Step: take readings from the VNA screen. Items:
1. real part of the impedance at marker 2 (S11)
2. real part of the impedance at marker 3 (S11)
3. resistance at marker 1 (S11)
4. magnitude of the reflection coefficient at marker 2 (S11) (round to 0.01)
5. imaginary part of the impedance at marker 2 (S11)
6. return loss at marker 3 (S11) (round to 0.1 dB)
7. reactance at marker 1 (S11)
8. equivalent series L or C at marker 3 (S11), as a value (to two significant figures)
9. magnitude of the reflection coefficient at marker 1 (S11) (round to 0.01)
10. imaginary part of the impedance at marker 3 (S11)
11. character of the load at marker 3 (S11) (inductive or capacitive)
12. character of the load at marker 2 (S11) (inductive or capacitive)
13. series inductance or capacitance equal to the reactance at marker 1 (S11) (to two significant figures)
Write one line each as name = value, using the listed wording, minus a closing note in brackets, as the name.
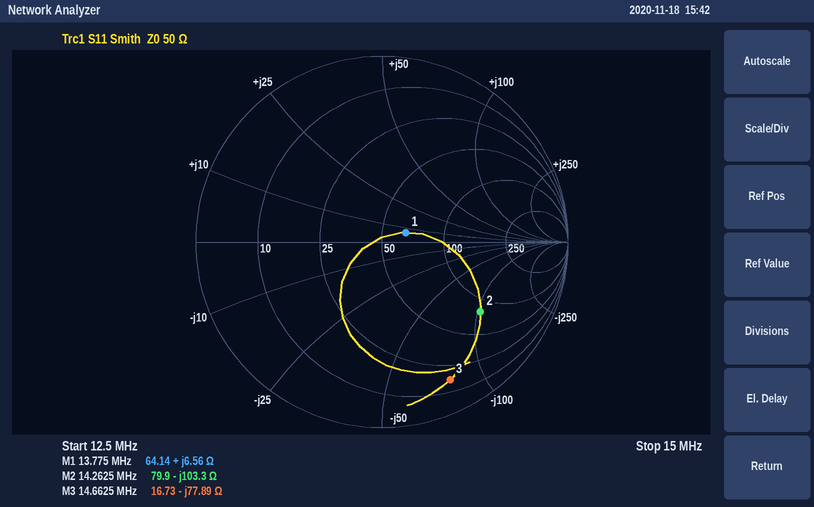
real part of the impedance at marker 2 = 79.9 Ω
real part of the impedance at marker 3 = 16.73 Ω
resistance at marker 1 = 64.14 Ω
magnitude of the reflection coefficient at marker 2 (S11) = 0.65
imaginary part of the impedance at marker 2 = -103.3 Ω
return loss at marker 3 (S11) = 1.7 dB
reactance at marker 1 = +6.56 Ω
equivalent series L or C at marker 3 (S11), as a value = 140 pF
magnitude of the reflection coefficient at marker 1 (S11) = 0.14
imaginary part of the impedance at marker 3 = -77.89 Ω
character of the load at marker 3 (S11) = capacitive
character of the load at marker 2 (S11) = capacitive
series inductance or capacitance equal to the reactance at marker 1 (S11) = 76 nH
